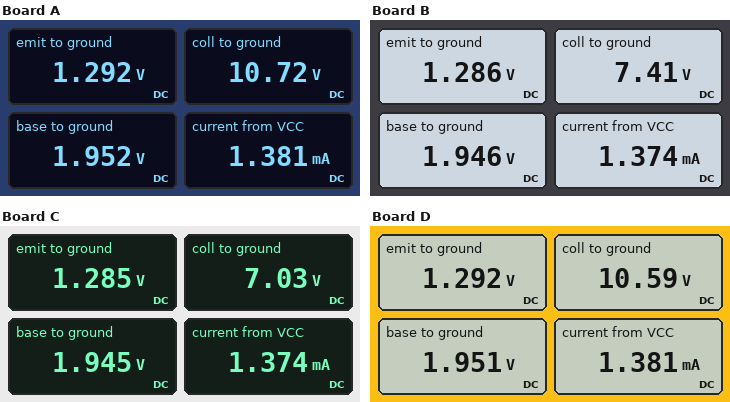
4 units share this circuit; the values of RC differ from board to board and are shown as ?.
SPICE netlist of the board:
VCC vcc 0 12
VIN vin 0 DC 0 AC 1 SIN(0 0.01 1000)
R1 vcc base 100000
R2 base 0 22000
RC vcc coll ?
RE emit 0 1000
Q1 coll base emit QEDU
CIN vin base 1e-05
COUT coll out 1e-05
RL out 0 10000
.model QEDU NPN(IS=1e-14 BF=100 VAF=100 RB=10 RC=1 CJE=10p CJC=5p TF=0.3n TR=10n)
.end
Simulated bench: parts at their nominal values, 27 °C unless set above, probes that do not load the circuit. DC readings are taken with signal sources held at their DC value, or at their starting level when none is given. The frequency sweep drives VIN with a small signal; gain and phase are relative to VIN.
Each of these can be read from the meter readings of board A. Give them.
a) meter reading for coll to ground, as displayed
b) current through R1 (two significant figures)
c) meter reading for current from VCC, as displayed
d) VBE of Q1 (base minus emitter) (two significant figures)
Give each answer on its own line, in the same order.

10.72 V
100 µA
1.381 mA
660 mV
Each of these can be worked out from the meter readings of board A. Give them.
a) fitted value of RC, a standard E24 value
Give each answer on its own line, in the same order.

1 kΩ
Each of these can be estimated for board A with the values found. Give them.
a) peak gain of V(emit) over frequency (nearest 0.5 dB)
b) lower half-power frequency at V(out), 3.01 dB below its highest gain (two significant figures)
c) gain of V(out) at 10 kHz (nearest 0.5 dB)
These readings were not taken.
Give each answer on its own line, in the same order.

0 dB
3.2 Hz
-1.0 dB
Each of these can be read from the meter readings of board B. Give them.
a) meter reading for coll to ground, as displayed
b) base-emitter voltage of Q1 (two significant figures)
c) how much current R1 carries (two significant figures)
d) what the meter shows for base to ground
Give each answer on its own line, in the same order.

7.41 V
660 mV
100 µA
1.946 V
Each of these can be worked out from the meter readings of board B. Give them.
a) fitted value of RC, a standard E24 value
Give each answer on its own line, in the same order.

3.6 kΩ
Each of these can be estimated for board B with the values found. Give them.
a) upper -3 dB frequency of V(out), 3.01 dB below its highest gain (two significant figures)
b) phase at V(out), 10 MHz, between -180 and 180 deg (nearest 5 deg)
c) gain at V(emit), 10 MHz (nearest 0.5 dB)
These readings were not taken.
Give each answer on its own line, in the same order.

31 MHz
145 deg
0 dB
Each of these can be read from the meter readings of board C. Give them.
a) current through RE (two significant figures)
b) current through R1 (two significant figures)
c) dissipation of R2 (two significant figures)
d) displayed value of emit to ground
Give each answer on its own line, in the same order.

1.3 mA
100 µA
170 µW
1.285 V
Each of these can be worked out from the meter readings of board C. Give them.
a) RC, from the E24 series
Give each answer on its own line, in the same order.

3.9 kΩ
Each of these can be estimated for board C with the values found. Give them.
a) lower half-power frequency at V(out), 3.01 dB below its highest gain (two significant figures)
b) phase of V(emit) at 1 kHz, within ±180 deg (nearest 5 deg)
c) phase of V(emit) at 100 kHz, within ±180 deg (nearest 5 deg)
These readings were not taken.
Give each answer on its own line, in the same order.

1.7 Hz
0 deg
0 deg
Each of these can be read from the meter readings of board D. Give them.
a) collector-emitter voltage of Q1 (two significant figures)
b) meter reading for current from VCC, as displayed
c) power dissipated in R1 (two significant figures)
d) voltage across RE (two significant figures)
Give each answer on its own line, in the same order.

9.3 V
1.381 mA
1.0 mW
1.3 V
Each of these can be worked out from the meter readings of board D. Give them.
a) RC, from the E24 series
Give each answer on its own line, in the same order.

1.1 kΩ
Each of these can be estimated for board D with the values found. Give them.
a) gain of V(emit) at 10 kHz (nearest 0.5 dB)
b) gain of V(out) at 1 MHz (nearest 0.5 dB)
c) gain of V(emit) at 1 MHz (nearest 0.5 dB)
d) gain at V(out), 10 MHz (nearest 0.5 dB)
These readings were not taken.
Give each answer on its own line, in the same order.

0 dB
-0.5 dB
0 dB
-0.5 dB
